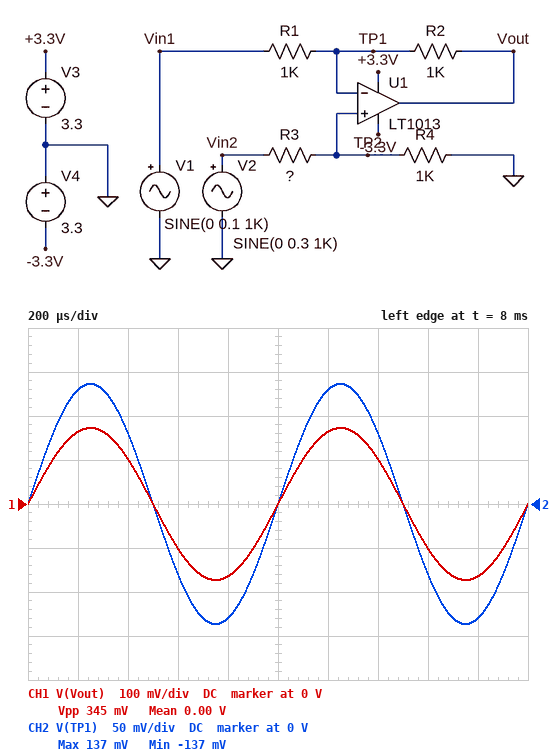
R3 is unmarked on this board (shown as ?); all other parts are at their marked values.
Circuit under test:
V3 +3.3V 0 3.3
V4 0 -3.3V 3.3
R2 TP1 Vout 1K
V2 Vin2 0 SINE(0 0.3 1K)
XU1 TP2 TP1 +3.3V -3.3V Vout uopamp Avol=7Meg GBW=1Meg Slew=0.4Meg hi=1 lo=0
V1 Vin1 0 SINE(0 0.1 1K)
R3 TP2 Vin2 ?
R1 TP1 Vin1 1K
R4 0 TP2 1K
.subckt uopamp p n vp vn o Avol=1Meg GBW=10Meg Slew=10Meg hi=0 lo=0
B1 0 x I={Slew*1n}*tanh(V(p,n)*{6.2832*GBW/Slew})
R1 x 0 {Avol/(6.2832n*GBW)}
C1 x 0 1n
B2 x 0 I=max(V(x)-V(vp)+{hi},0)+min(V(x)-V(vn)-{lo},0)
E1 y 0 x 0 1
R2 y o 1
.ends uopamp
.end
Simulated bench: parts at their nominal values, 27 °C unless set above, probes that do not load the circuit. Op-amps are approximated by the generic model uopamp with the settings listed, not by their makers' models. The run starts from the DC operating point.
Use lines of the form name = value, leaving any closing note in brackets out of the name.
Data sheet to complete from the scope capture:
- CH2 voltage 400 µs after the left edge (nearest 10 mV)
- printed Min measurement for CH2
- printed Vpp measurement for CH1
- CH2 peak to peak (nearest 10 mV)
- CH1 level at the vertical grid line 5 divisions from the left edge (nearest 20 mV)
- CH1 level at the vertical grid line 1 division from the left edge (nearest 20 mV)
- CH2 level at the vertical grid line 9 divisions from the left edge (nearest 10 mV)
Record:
CH2 voltage 400 µs after the left edge = 80 mV
printed Min measurement for CH2 = -137 mV
printed Vpp measurement for CH1 = 345 mV
CH2 peak to peak = 270 mV
CH1 level at the vertical grid line 5 divisions from the left edge = 0 V
CH1 level at the vertical grid line 1 division from the left edge = 160 mV
CH2 level at the vertical grid line 9 divisions from the left edge = -130 mV
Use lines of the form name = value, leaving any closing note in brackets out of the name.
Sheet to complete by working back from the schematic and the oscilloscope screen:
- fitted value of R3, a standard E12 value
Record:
fitted value of R3, a standard E12 value = 1.2 kΩ
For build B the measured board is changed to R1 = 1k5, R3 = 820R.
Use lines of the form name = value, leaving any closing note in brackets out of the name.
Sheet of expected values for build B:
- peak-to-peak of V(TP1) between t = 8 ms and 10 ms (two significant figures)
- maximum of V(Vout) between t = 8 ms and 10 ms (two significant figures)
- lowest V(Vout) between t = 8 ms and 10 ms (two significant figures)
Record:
peak-to-peak of V(TP1) between t = 8 ms and 10 ms = 330 mV
maximum of V(Vout) between t = 8 ms and 10 ms = 210 mV
lowest V(Vout) between t = 8 ms and 10 ms = -210 mV
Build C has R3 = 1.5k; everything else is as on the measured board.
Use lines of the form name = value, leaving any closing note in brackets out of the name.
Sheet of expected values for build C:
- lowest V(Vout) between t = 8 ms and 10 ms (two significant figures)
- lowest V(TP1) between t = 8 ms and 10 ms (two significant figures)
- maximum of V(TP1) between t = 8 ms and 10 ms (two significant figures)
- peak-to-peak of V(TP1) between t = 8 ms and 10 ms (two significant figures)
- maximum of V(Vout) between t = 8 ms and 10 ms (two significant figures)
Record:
lowest V(Vout) between t = 8 ms and 10 ms = -140 mV
lowest V(TP1) between t = 8 ms and 10 ms = -120 mV
maximum of V(TP1) between t = 8 ms and 10 ms = 120 mV
peak-to-peak of V(TP1) between t = 8 ms and 10 ms = 240 mV
maximum of V(Vout) between t = 8 ms and 10 ms = 140 mV
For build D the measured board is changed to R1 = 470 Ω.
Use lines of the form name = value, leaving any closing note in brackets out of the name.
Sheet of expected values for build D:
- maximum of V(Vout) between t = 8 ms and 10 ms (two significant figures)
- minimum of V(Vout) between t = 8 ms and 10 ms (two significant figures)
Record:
maximum of V(Vout) between t = 8 ms and 10 ms = 210 mV
minimum of V(Vout) between t = 8 ms and 10 ms = -210 mV
